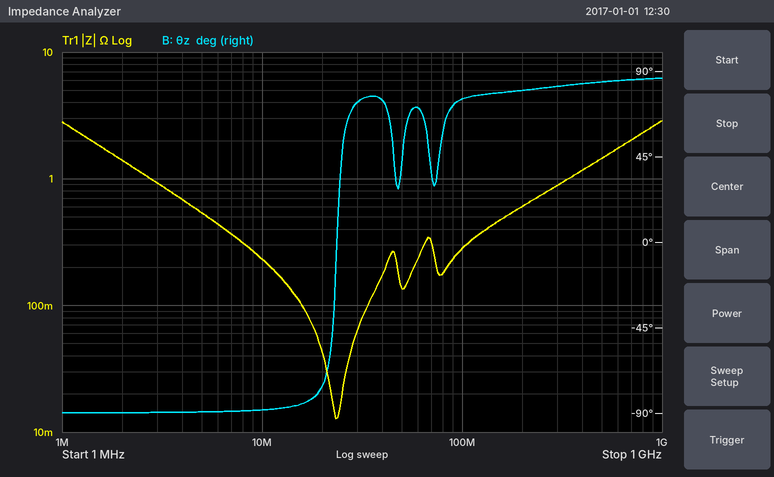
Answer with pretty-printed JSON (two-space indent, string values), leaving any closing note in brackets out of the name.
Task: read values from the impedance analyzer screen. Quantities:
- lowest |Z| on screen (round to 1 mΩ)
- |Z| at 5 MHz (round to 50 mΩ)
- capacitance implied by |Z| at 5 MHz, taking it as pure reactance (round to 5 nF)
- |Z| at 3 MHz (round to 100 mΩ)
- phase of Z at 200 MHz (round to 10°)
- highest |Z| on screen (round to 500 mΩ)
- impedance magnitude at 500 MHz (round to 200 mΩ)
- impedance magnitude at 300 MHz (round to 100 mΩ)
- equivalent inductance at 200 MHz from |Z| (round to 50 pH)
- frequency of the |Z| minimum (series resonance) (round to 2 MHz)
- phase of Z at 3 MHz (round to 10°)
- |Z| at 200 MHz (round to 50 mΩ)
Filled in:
{
  "lowest |Z| on screen": "13 mΩ",
  "|Z| at 5 MHz": "550 mΩ",
  "capacitance implied by |Z| at 5 MHz, taking it as pure reactance": "60 nF",
  "|Z| at 3 MHz": "900 mΩ",
  "phase of Z at 200 MHz": "80°",
  "highest |Z| on screen": "3.0 Ω",
  "impedance magnitude at 500 MHz": "1.4 Ω",
  "impedance magnitude at 300 MHz": "900 mΩ",
  "equivalent inductance at 200 MHz from |Z|": "500 pH",
  "frequency of the |Z| minimum (series resonance)": "24 MHz",
  "phase of Z at 3 MHz": "-90°",
  "|Z| at 200 MHz": "600 mΩ"
}
